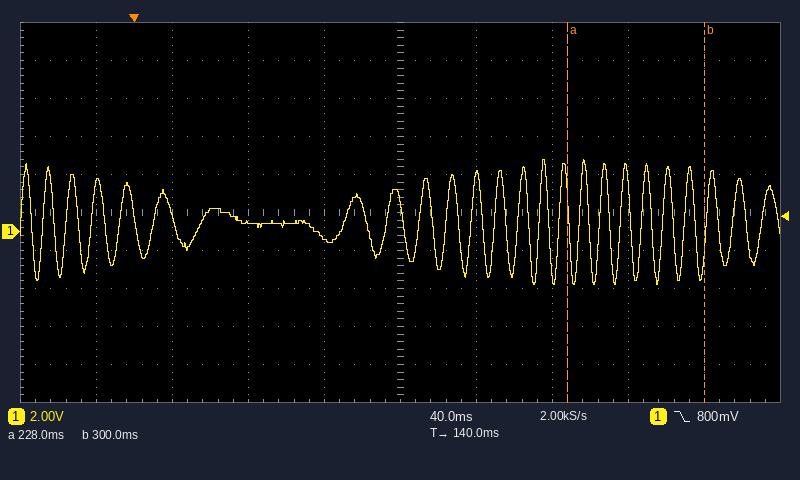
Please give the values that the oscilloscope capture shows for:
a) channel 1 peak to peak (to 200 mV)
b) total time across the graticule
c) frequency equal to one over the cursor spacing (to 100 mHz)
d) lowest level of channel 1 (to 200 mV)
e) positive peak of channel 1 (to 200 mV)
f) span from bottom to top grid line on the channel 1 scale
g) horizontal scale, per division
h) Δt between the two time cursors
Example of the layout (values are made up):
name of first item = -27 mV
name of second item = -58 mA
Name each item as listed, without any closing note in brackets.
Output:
channel 1 peak to peak = 6.6 V
total time across the graticule = 400 ms
frequency equal to one over the cursor spacing = 13.9 Hz
lowest level of channel 1 = -2.8 V
positive peak of channel 1 = 3.8 V
span from bottom to top grid line on the channel 1 scale = 20 V
horizontal scale, per division = 40 ms
Δt between the two time cursors = 72 ms
